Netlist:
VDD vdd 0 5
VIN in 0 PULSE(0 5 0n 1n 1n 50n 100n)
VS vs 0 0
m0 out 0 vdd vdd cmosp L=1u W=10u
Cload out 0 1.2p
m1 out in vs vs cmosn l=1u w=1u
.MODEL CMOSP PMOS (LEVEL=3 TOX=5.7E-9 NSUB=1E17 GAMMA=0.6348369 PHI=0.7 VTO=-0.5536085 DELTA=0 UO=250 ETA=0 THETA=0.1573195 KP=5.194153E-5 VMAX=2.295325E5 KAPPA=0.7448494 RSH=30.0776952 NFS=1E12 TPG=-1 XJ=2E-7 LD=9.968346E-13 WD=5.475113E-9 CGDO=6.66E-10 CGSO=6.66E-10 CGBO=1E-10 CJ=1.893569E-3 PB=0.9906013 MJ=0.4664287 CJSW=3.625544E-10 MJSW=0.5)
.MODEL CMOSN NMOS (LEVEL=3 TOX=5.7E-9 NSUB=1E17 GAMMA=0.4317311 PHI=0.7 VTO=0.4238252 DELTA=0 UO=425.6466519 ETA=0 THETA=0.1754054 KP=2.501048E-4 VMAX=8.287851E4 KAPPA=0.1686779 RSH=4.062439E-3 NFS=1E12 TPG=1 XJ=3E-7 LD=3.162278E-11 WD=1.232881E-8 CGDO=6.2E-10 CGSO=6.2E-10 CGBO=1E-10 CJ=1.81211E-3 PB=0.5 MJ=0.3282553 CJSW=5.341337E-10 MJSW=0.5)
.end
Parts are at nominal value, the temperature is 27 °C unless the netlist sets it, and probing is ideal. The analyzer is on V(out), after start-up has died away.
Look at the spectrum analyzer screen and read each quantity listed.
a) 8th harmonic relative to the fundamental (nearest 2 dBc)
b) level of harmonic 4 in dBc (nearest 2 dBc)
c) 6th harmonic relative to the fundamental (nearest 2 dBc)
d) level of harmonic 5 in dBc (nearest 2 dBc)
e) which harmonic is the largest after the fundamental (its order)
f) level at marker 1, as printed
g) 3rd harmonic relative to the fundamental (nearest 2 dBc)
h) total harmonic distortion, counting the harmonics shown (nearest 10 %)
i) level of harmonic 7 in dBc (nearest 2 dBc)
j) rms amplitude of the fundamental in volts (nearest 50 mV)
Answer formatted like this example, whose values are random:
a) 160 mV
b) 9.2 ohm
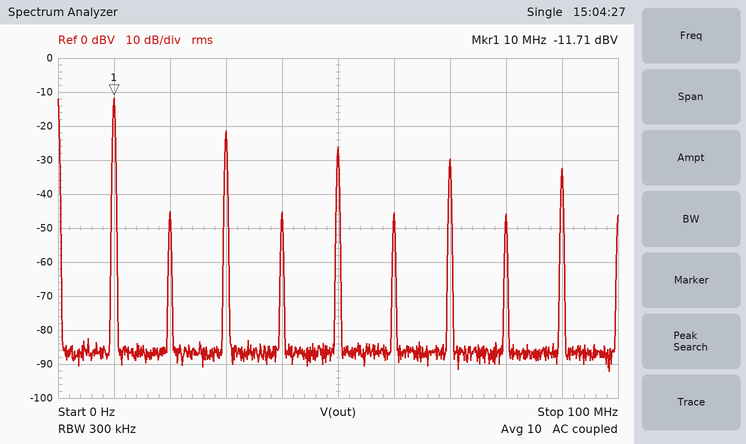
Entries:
a) -34 dBc
b) -34 dBc
c) -34 dBc
d) -14 dBc
e) 3
f) -11.71 dBV
g) -10 dBc
h) 40 %
i) -18 dBc
j) 250 mV
